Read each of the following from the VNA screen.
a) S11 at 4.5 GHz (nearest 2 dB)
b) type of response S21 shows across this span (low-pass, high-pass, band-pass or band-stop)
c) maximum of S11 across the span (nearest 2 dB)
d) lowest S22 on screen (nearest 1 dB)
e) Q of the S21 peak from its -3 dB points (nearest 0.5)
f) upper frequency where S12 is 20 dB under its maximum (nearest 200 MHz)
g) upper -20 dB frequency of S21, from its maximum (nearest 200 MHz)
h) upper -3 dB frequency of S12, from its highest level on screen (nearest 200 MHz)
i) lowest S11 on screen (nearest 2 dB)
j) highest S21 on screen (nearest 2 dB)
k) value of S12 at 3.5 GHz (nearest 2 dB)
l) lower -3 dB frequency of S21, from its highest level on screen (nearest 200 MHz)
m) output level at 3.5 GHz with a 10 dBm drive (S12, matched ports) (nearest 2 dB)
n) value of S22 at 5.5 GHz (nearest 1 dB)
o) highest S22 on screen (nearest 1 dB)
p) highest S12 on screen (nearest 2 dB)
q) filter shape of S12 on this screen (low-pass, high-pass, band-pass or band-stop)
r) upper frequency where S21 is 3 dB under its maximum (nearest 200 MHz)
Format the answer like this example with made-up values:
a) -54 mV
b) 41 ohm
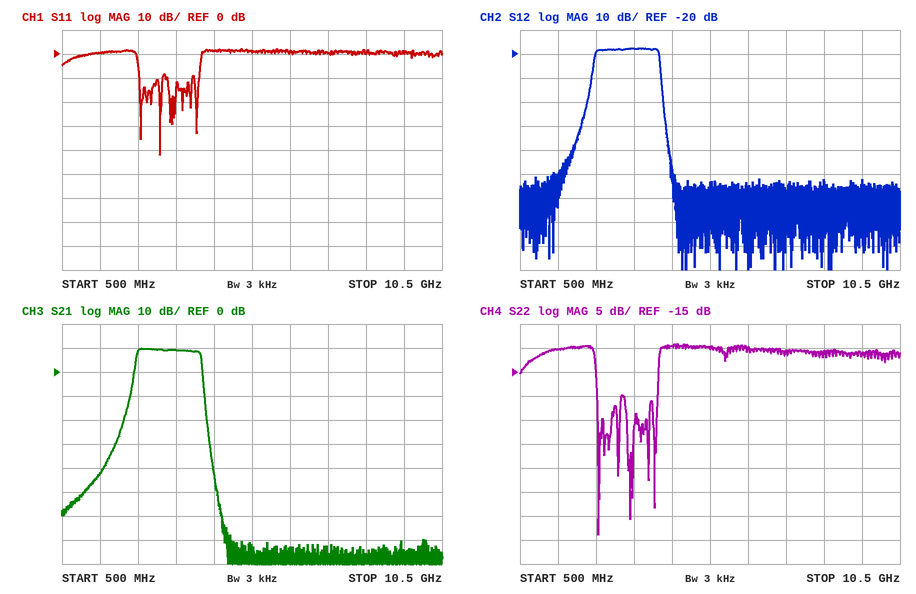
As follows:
a) 2 dB
b) band-pass
c) 2 dB
d) -49 dB
e) 2.0
f) 4.2 GHz
g) 4.2 GHz
h) 4.2 GHz
i) -42 dB
j) 10 dB
k) -18 dB
l) 2.4 GHz
m) -8 dBm
n) -10 dB
o) -9 dB
p) -18 dB
q) band-pass
r) 4.2 GHz
